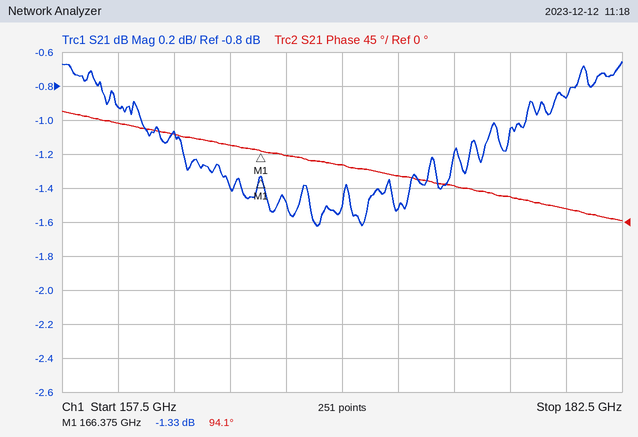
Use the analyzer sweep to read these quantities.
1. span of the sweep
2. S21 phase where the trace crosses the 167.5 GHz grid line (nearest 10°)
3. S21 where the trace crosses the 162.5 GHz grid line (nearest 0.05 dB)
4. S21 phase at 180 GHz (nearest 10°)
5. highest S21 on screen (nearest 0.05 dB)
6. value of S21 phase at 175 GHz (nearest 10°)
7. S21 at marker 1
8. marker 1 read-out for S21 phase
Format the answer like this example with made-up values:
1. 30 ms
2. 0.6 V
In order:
1. 25 GHz
2. 90°
3. -1.05 dB
4. 20°
5. -0.65 dB
6. 50°
7. -1.33 dB
8. 94.1°
